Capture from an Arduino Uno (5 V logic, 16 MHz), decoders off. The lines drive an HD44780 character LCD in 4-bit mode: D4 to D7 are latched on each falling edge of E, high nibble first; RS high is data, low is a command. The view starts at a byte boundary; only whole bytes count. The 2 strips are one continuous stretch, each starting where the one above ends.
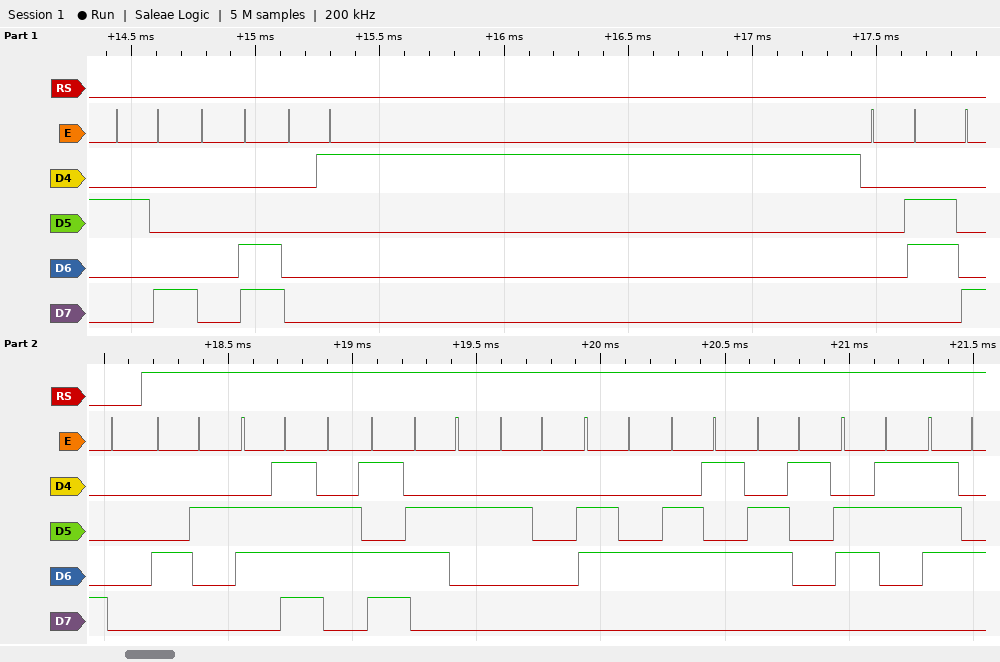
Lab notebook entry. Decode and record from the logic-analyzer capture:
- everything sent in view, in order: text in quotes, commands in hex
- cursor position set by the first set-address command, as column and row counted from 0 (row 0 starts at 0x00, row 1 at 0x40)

0x28 0x0C 0x01 0x06 0x80 "Bomb deact"
column 0, row 0
